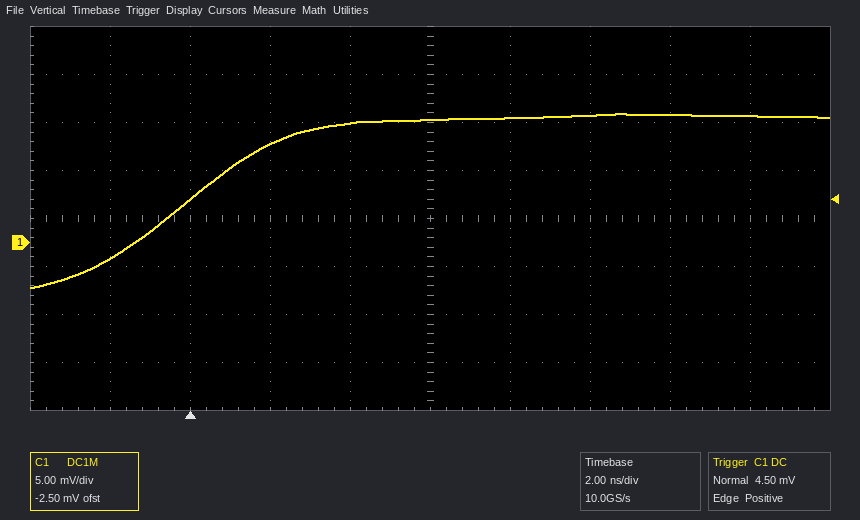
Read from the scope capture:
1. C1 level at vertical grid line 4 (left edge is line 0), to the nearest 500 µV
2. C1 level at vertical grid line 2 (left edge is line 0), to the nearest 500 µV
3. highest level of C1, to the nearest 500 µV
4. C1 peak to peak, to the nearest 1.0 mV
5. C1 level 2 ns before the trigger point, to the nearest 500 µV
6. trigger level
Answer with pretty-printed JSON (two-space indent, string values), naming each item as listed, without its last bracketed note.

{
  "C1 level at vertical grid line 4 (left edge is line 0), to the nearest 500 µV": "12.5 mV",
  "C1 level at vertical grid line 2 (left edge is line 0), to the nearest 500 µV": "4.5 mV",
  "highest level of C1, to the nearest 500 µV": "13.5 mV",
  "C1 peak to peak, to the nearest 1.0 mV": "18.0 mV",
  "C1 level 2 ns before the trigger point, to the nearest 500 µV": "-1.5 mV",
  "trigger level": "4.50 mV"
}
